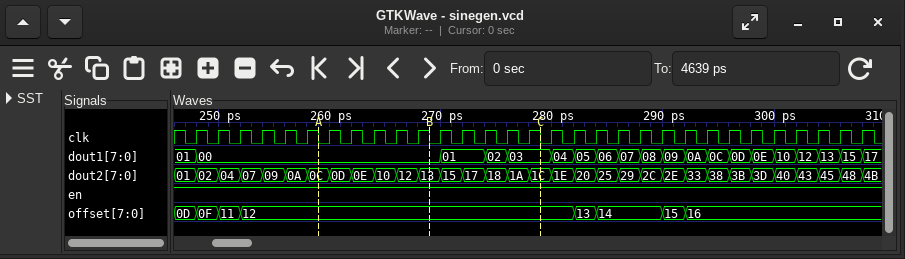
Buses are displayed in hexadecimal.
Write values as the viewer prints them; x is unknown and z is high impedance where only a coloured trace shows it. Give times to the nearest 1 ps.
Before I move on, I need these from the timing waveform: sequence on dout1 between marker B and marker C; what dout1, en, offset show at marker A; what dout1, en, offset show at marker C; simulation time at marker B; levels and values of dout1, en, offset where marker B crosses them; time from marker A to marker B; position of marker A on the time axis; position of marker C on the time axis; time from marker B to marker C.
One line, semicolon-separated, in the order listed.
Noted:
00, 01, 02, 03; dout1=00, en=1, offset=12; dout1=03, en=1, offset=12; 269 ps; dout1=00, en=1, offset=12; 10 ps; 259 ps; 279 ps; 10 ps
